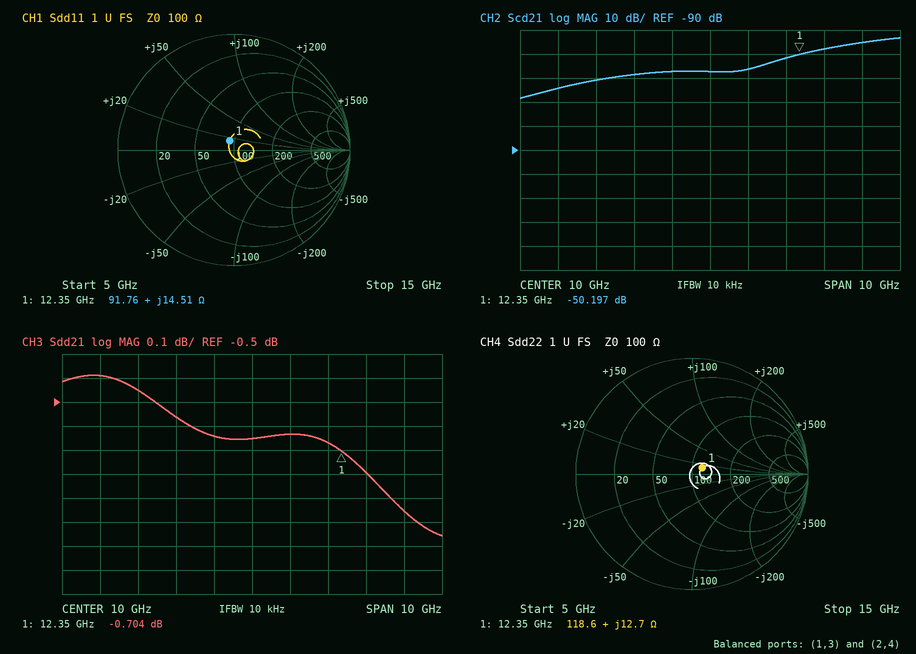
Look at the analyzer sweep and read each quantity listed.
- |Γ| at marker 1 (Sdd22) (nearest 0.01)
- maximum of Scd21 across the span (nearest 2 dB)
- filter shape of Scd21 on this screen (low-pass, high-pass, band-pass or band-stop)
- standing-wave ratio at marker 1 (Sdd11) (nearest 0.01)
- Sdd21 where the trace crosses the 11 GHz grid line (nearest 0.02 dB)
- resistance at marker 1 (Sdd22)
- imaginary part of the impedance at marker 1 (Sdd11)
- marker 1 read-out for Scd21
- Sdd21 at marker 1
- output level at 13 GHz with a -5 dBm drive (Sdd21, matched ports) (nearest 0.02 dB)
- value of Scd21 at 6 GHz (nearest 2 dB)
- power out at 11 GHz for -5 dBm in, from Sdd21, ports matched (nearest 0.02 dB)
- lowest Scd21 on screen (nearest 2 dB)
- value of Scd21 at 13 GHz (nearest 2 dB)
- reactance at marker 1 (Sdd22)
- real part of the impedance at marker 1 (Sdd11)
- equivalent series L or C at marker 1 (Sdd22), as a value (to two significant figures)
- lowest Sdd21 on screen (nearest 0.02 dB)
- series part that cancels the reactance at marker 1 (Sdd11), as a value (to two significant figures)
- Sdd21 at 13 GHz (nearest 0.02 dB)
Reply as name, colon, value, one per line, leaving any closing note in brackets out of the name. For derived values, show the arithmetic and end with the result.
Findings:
|Γ| at marker 1 (Sdd22): 0.10
maximum of Scd21 across the span: -44 dB
filter shape of Scd21 on this screen: high-pass
standing-wave ratio at marker 1 (Sdd11): 1.19
Sdd21 where the trace crosses the 11 GHz grid line: -0.64 dB
resistance at marker 1: 118.6 Ω
imaginary part of the impedance at marker 1: +14.51 Ω
marker 1 read-out for Scd21: -50.197 dB
Sdd21 at marker 1: -0.704 dB
output level at 13 GHz with a -5 dBm drive (Sdd21, matched ports): -5 dBm + (-0.80 dB) = -5.80 dBm
value of Scd21 at 6 GHz: -64 dB
power out at 11 GHz for -5 dBm in, from Sdd21, ports matched: -5 dBm + (-0.64 dB) = -5.64 dBm
lowest Scd21 on screen: -68 dB
value of Scd21 at 13 GHz: -48 dB
reactance at marker 1: +12.7 Ω
real part of the impedance at marker 1: 91.76 Ω
equivalent series L or C at marker 1 (Sdd22), as a value: L = 12.7 Ω/(2π × 12.35 GHz) ≈ 164 pH, so 160 pH to two significant figures
lowest Sdd21 on screen: -1.06 dB
series part that cancels the reactance at marker 1 (Sdd11), as a value: C = 1/(2π × 12.35 GHz × 14.51 Ω) ≈ 888 fF, so 890 fF to two significant figures
Sdd21 at 13 GHz: -0.80 dB
